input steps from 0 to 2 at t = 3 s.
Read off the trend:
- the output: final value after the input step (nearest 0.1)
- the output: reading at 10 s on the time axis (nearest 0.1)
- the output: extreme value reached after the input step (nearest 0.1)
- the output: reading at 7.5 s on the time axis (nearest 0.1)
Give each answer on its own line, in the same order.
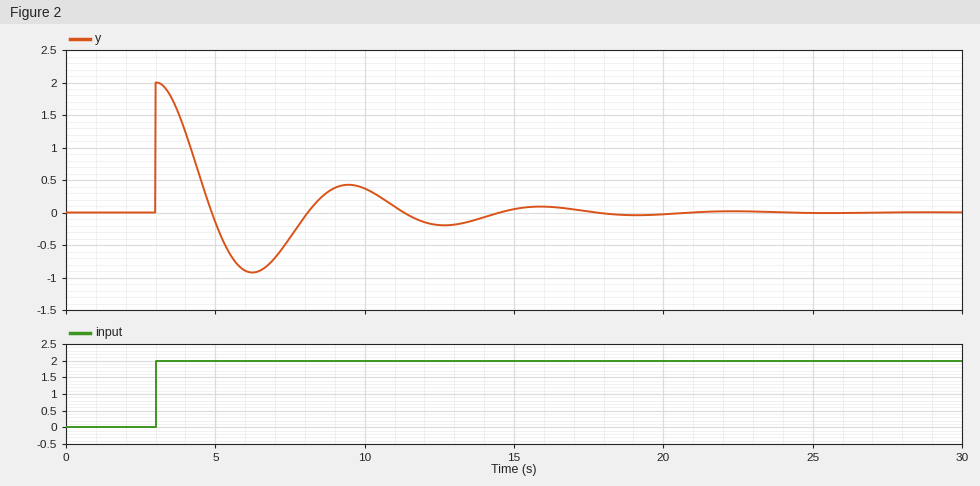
0.0
0.4
2.0
-0.4
